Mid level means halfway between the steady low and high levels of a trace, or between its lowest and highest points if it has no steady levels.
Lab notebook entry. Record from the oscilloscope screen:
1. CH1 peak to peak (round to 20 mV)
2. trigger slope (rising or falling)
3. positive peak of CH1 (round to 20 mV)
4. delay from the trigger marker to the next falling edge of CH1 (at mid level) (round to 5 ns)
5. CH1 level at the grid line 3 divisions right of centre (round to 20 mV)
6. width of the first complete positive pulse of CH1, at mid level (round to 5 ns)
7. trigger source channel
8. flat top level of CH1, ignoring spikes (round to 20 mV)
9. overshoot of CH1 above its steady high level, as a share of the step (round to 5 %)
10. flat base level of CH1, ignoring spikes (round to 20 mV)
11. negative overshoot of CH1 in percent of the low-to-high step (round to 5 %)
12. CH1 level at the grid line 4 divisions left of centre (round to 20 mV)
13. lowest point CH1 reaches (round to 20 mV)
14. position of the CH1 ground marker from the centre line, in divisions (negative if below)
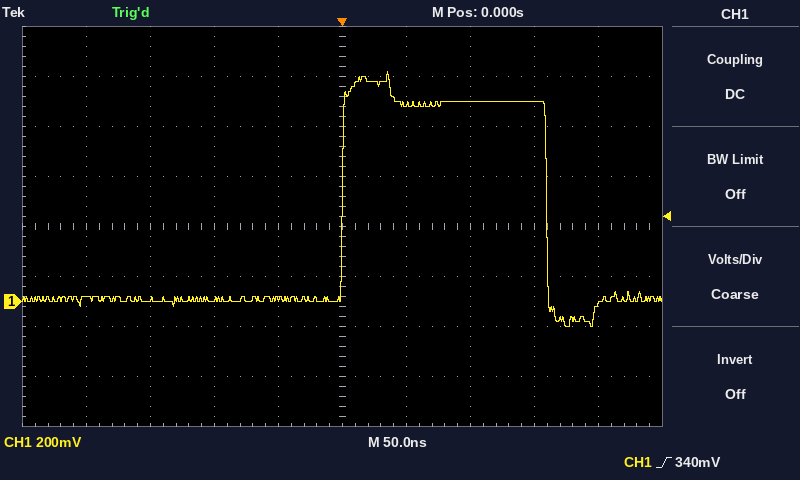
1.02 V
rising
920 mV
160 ns
800 mV
160 ns
CH1
800 mV
15 %
0 mV
15 %
20 mV
-100 mV
-1.5 div
